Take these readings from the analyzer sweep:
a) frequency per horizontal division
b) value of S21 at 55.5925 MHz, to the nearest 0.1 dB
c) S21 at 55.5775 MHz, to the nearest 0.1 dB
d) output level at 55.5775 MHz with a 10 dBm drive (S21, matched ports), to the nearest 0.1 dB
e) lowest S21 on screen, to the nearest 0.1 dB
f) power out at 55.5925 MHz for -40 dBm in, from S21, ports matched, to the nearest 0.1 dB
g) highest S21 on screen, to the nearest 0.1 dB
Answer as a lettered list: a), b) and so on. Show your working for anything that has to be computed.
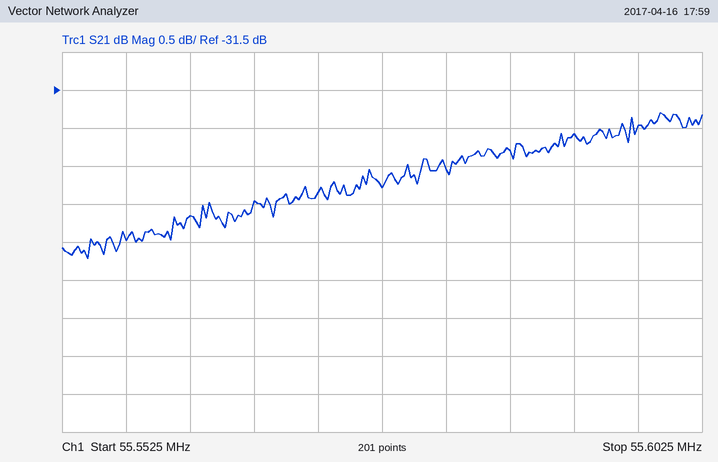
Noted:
a) 5 kHz
b) -32.1 dB
c) -32.8 dB
d) 10 dBm + (-32.8 dB) = -22.8 dBm
e) -33.7 dB
f) -40 dBm + (-32.1 dB) = -72.1 dBm
g) -31.8 dB
